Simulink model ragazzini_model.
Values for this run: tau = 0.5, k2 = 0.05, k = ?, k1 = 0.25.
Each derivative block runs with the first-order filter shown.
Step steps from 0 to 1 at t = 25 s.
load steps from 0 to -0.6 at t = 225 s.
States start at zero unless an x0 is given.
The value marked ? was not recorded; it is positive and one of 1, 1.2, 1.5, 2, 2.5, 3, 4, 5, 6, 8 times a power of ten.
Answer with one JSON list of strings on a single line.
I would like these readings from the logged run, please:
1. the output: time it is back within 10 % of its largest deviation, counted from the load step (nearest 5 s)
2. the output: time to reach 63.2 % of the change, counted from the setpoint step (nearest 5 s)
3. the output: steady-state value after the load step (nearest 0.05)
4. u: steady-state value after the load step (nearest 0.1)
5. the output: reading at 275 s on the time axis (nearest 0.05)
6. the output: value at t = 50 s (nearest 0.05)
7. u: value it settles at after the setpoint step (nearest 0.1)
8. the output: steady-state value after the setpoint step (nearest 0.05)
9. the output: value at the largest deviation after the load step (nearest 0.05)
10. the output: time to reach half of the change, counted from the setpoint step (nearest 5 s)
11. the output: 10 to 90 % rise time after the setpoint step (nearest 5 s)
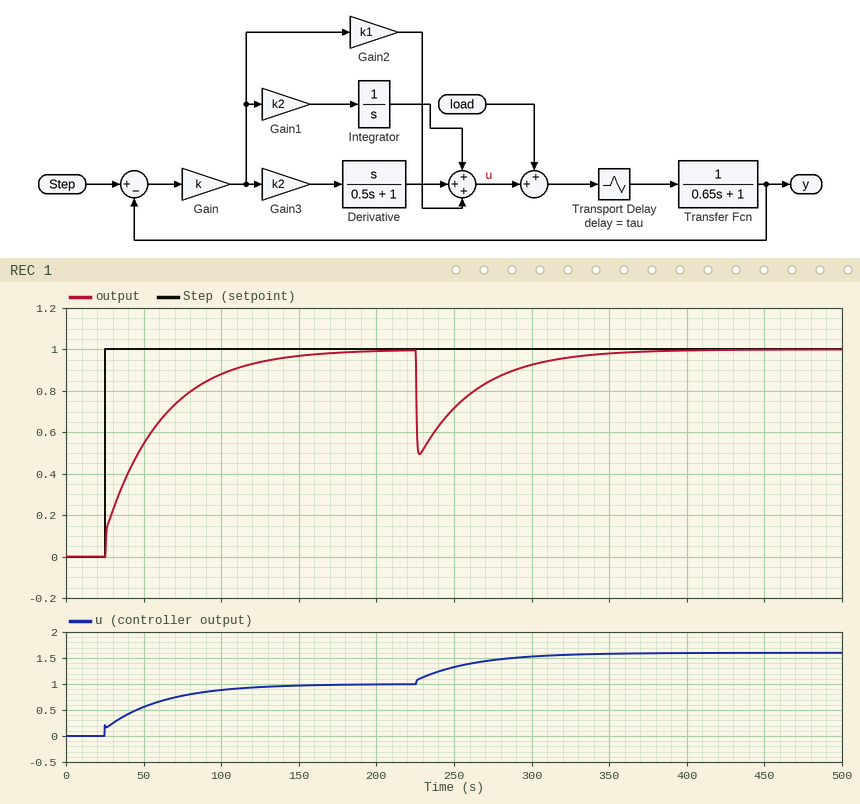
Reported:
["90 s", "35 s", "1.00", "1.6", "0.85", "0.55", "1.0", "1.00", "0.50", "20 s", "80 s"]
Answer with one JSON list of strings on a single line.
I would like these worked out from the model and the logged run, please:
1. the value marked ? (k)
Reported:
["0.6"]
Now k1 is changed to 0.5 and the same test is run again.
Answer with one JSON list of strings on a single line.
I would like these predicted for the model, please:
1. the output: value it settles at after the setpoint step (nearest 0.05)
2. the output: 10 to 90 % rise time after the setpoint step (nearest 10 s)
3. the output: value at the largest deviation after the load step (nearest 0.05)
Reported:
["1.00", "90 s", "0.55"]
